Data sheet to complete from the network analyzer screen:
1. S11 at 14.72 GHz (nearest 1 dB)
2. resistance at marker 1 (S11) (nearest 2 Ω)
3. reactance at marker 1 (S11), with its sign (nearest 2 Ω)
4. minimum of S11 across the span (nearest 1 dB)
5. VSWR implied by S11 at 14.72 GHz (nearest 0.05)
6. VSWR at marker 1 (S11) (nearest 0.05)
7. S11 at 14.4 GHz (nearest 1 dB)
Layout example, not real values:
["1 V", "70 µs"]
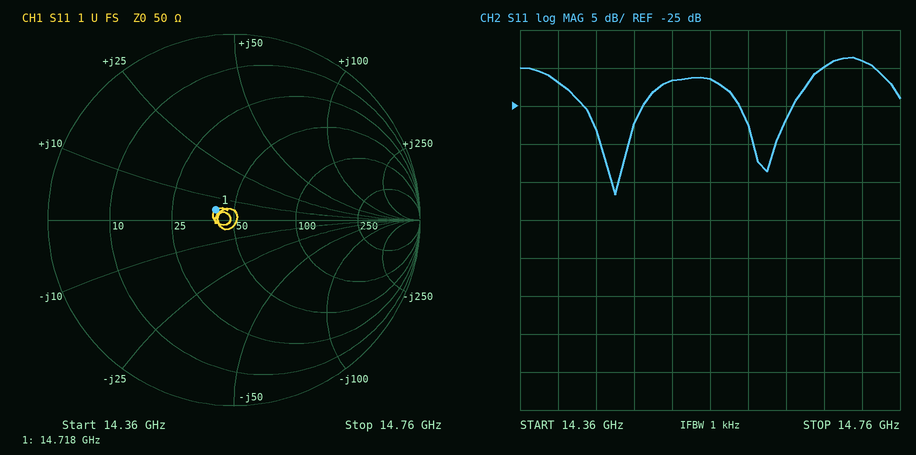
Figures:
["-19 dB", "40 Ω", "+4 Ω", "-37 dB", "1.25", "1.25", "-22 dB"]
